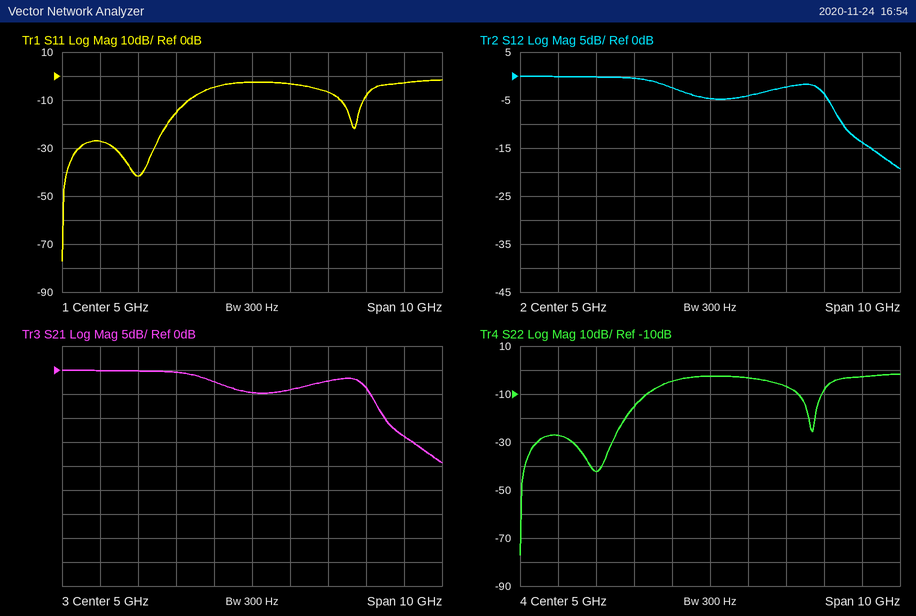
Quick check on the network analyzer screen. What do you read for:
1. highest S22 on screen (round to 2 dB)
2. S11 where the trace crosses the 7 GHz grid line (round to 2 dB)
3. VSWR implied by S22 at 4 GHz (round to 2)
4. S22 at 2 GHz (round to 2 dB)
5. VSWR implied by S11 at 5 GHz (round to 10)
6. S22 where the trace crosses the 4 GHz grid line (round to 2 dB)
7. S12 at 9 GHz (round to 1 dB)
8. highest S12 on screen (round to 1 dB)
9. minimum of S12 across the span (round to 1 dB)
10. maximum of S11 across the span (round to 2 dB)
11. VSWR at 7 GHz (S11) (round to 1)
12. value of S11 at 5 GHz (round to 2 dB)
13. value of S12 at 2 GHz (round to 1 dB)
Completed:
-2 dB
-6 dB
4
-42 dB
10
-4 dB
-14 dB
0 dB
-19 dB
-2 dB
3
-2 dB
0 dB
